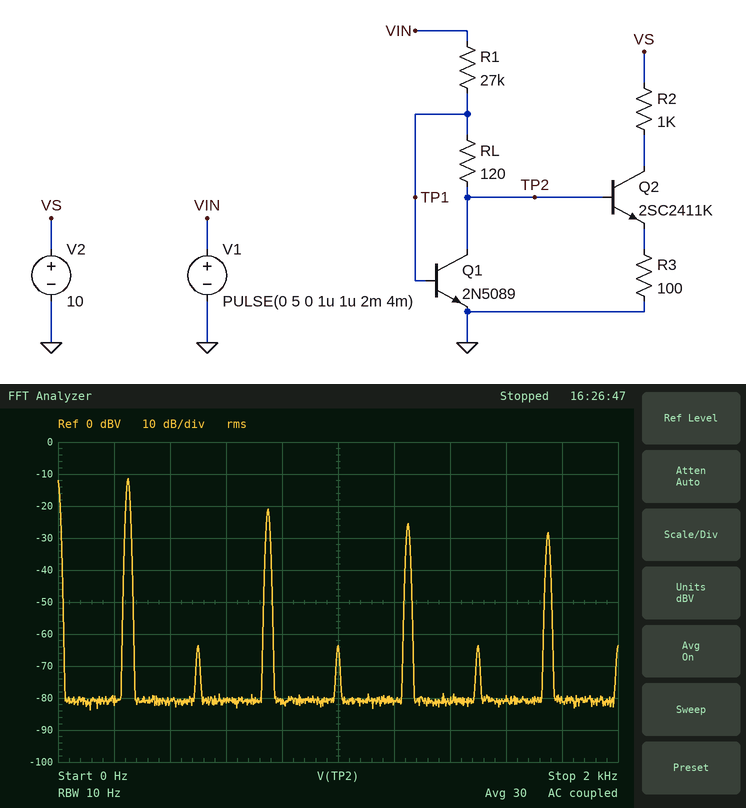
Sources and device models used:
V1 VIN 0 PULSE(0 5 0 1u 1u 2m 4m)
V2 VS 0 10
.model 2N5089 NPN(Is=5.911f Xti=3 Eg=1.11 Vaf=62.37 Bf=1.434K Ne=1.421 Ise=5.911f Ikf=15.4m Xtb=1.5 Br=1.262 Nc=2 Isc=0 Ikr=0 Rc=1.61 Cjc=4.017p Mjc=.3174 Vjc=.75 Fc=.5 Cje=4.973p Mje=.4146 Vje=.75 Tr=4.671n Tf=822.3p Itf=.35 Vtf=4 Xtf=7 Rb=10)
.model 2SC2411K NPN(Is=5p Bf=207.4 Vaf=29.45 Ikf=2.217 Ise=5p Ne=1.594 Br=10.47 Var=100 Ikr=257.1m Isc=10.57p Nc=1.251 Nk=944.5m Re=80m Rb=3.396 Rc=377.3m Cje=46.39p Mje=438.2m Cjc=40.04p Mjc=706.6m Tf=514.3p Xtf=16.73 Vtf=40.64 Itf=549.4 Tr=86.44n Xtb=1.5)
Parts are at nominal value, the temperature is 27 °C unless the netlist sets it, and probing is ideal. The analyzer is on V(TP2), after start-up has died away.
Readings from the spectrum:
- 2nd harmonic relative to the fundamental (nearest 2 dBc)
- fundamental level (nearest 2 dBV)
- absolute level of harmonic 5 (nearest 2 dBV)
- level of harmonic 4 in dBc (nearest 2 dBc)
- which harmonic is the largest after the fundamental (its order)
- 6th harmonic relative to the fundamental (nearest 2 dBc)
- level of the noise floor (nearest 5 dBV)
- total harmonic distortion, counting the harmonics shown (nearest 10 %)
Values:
-52 dBc
-12 dBV
-26 dBV
-52 dBc
3
-52 dBc
-80 dBV
40 %
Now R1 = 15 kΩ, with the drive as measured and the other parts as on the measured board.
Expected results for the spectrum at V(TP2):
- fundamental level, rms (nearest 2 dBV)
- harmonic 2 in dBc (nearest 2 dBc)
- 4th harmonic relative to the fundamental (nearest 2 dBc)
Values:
-12 dBV
-54 dBc
-54 dBc
